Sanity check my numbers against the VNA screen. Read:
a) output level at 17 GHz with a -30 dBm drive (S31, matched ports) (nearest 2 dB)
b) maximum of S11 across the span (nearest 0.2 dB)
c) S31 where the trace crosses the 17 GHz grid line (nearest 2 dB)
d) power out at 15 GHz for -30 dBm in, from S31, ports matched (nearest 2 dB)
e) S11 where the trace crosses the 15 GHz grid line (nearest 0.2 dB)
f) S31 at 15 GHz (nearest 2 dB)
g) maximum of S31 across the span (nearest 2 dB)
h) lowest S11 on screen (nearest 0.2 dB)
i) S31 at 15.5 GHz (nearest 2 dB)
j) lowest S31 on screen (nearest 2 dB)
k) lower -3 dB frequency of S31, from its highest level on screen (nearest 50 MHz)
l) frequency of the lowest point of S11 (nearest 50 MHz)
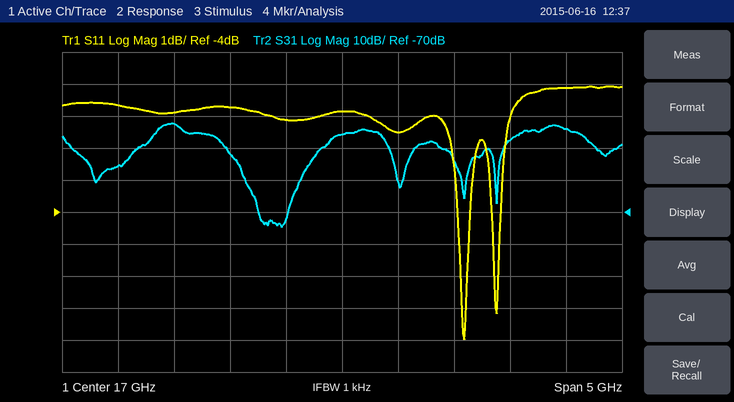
-76 dBm
0.0 dB
-46 dB
-86 dBm
-0.6 dB
-56 dB
-42 dB
-8.0 dB
-42 dB
-74 dB
15.35 GHz
18.10 GHz
